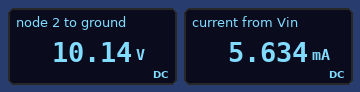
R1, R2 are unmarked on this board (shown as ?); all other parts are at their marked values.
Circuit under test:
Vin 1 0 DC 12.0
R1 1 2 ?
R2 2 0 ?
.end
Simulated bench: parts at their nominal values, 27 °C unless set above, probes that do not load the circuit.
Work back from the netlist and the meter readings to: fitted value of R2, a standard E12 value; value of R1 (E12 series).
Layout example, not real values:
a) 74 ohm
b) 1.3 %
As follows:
a) 1.8 kΩ
b) 330 Ω
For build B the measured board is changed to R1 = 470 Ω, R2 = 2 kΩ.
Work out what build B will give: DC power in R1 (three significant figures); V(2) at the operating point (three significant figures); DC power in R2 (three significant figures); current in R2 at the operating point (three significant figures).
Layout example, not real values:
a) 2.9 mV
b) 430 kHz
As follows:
a) 11.1 mW
b) 9.72 V
c) 47.2 mW
d) 4.86 mA
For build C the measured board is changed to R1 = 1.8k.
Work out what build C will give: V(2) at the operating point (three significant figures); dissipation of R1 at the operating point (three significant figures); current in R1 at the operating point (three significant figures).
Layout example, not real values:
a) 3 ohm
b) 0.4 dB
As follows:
a) 6.00 V
b) 20.0 mW
c) 3.33 mA
